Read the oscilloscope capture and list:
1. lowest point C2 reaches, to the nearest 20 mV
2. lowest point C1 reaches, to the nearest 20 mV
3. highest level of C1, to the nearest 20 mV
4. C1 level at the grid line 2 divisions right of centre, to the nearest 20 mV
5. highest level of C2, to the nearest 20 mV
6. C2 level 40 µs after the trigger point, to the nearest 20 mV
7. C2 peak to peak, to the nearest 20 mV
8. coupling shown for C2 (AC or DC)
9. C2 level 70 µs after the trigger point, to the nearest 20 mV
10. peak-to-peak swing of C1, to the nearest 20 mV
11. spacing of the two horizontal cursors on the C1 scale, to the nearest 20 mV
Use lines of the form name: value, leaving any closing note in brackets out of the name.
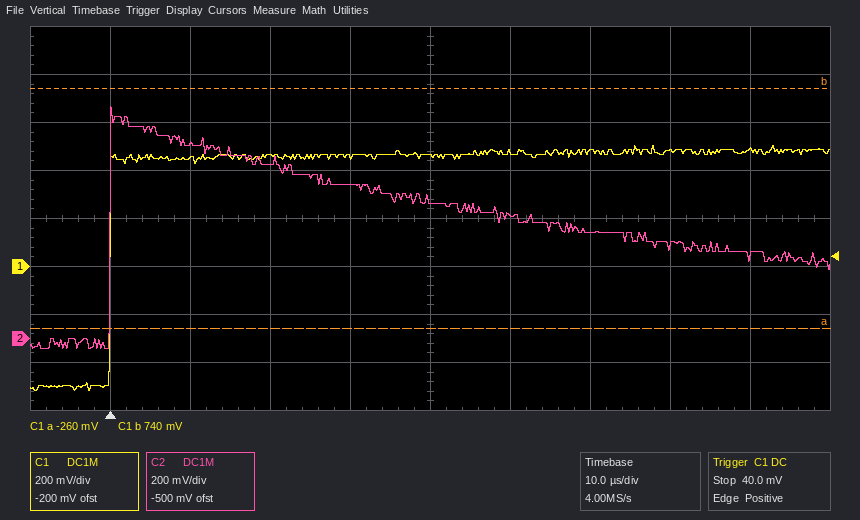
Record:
lowest point C2 reaches, to the nearest 20 mV: -40 mV
lowest point C1 reaches, to the nearest 20 mV: -520 mV
highest level of C1, to the nearest 20 mV: 500 mV
C1 level at the grid line 2 divisions right of centre, to the nearest 20 mV: 480 mV
highest level of C2, to the nearest 20 mV: 960 mV
C2 level 40 µs after the trigger point, to the nearest 20 mV: 580 mV
C2 peak to peak, to the nearest 20 mV: 1.00 V
coupling shown for C2: DC
C2 level 70 µs after the trigger point, to the nearest 20 mV: 380 mV
peak-to-peak swing of C1, to the nearest 20 mV: 1.02 V
spacing of the two horizontal cursors on the C1 scale, to the nearest 20 mV: 1.00 V
